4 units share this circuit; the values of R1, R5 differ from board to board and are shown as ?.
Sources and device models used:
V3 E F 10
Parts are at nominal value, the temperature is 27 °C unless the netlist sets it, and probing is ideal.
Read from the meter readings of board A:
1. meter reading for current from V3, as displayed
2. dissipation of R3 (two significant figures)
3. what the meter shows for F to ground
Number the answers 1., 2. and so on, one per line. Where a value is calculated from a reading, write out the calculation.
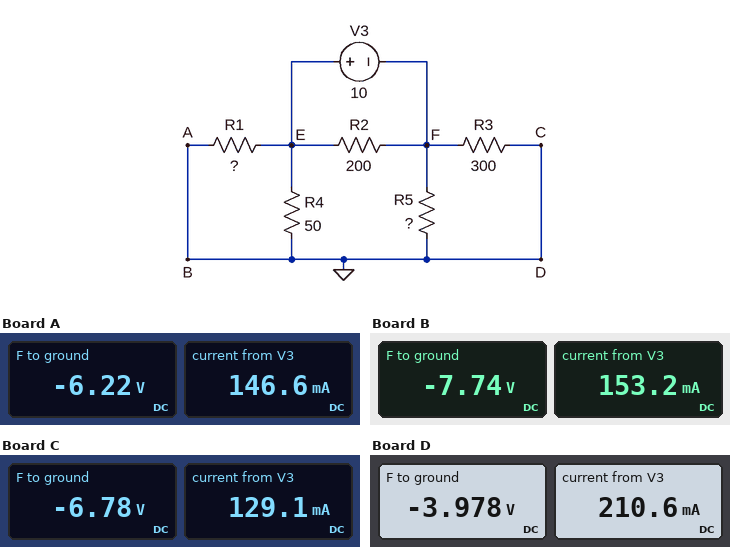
1. 146.6 mA
2. (0 V - (-6.22 V))^2 / 300 Ω = 130 mW
3. -6.22 V
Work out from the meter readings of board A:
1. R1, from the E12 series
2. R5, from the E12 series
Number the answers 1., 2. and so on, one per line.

1. 180 Ω
2. 82 Ω
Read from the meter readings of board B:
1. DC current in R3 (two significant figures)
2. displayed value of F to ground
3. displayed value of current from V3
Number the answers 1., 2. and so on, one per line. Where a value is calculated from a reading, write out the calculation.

1. (0 V - (-7.74 V)) / 300 Ω = 26 mA
2. -7.74 V
3. 153.2 mA
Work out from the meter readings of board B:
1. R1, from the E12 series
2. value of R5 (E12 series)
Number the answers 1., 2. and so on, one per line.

1. 39 Ω
2. 100 Ω
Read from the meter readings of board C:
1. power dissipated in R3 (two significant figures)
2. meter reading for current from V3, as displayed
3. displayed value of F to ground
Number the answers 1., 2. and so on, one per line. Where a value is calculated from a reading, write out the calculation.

1. (0 V - (-6.78 V))^2 / 300 Ω = 150 mW
2. 129.1 mA
3. -6.78 V
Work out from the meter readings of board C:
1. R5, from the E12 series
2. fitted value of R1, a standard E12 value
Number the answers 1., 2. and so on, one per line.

1. 120 Ω
2. 220 Ω
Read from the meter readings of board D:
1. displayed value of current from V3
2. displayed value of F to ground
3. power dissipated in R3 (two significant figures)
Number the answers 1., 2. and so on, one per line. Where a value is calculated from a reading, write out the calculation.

1. 210.6 mA
2. -3.978 V
3. (0 V - (-3.978 V))^2 / 300 Ω = 53 mW
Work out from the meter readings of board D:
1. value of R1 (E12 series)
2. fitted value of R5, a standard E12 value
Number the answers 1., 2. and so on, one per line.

1. 150 Ω
2. 27 Ω
